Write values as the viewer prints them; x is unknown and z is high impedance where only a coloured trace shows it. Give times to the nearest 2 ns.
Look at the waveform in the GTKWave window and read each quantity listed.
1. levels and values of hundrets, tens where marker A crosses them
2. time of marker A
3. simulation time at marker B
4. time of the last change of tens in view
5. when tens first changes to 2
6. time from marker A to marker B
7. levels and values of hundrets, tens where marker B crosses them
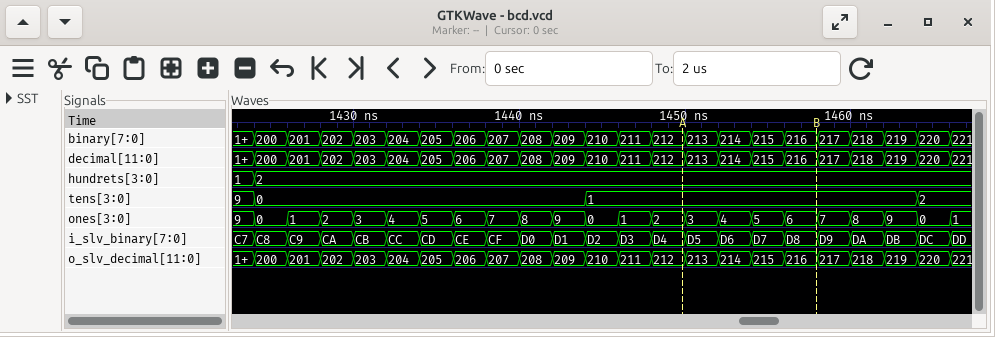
hundrets=2, tens=1
1450 ns
1458 ns
1464 ns
1464 ns
8 ns
hundrets=2, tens=1
